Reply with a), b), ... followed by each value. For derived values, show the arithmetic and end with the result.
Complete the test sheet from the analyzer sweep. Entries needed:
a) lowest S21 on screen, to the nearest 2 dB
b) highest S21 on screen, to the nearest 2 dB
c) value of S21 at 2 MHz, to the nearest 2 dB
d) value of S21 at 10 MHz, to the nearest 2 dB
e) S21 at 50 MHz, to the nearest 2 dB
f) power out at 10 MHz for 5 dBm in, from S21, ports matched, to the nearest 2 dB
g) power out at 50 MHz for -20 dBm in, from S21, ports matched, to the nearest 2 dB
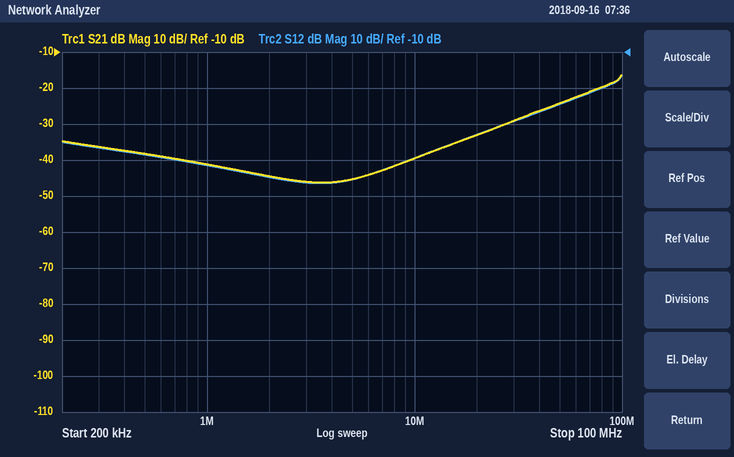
a) -46 dB
b) -16 dB
c) -44 dB
d) -40 dB
e) -24 dB
f) 5 dBm + (-40 dB) = -34 dBm
g) -20 dBm + (-24 dB) = -44 dBm
